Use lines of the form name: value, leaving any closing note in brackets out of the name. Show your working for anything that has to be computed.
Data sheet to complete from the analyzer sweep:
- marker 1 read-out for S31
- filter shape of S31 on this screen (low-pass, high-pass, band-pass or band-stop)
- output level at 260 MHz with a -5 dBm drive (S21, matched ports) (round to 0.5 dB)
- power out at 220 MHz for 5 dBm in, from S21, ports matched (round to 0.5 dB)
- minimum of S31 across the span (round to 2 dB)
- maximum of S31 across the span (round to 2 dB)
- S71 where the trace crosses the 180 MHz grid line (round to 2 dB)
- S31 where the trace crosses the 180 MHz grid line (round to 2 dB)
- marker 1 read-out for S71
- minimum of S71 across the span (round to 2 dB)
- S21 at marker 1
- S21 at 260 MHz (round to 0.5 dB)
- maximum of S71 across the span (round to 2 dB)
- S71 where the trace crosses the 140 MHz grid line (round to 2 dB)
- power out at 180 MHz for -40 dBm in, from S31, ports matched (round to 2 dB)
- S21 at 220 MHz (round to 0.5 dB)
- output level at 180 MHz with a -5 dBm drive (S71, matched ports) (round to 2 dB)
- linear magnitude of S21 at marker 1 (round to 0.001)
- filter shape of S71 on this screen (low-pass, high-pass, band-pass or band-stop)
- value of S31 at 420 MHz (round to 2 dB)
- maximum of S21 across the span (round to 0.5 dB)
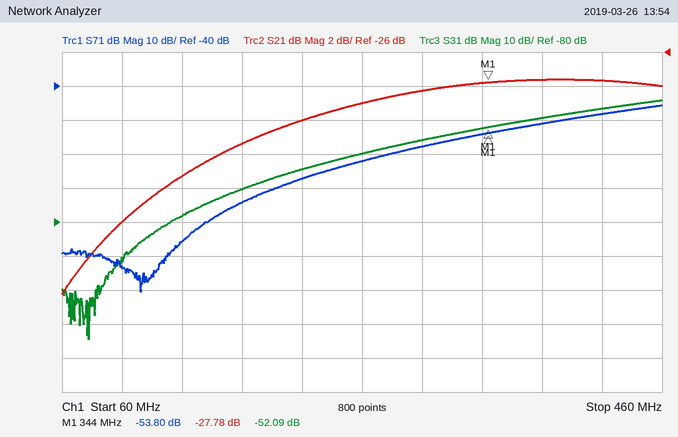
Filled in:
marker 1 read-out for S31: -52.09 dB
filter shape of S31 on this screen: high-pass
output level at 260 MHz with a -5 dBm drive (S21, matched ports): -5 dBm + (-29.0 dB) = -34.0 dBm
power out at 220 MHz for 5 dBm in, from S21, ports matched: 5 dBm + (-30.0 dB) = -25.0 dBm
minimum of S31 across the span: -114 dB
maximum of S31 across the span: -44 dB
S71 where the trace crosses the 180 MHz grid line: -74 dB
S31 where the trace crosses the 180 MHz grid line: -70 dB
marker 1 read-out for S71: -53.80 dB
minimum of S71 across the span: -100 dB
S21 at marker 1: -27.78 dB
S21 at 260 MHz: -29.0 dB
maximum of S71 across the span: -46 dB
S71 where the trace crosses the 140 MHz grid line: -86 dB
power out at 180 MHz for -40 dBm in, from S31, ports matched: -40 dBm + (-70 dB) = -110 dBm
S21 at 220 MHz: -30.0 dB
output level at 180 MHz with a -5 dBm drive (S71, matched ports): -5 dBm + (-74 dB) = -80 dBm
linear magnitude of S21 at marker 1: 10^(-27.78/20) ≈ 0.041
filter shape of S71 on this screen: high-pass
value of S31 at 420 MHz: -46 dB
maximum of S21 across the span: -27.5 dB
